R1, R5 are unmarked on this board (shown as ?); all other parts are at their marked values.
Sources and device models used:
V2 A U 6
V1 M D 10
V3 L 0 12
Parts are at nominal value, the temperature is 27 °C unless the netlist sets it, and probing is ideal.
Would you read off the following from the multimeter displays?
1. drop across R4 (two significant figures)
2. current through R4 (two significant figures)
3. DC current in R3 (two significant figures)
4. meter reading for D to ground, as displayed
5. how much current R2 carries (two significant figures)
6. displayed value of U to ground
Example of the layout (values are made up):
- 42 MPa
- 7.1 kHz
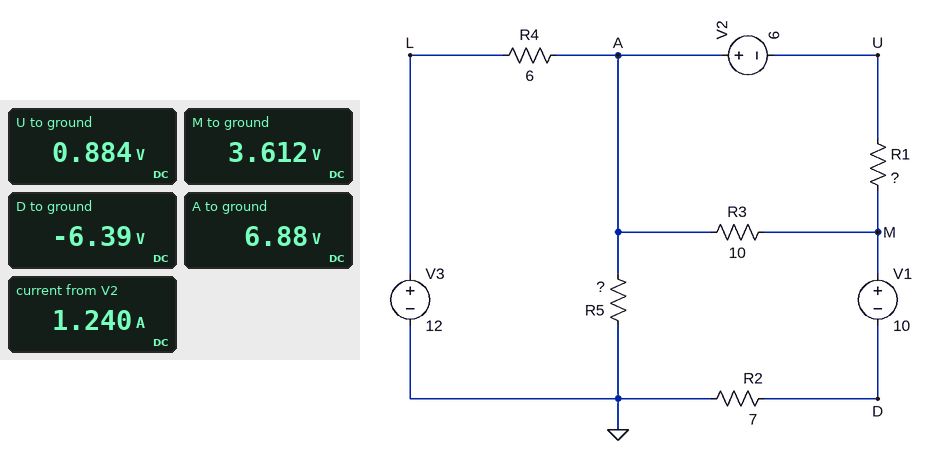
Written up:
- 5.1 V
- 850 mA
- 330 mA
- -6.39 V
- 910 mA
- 0.884 V
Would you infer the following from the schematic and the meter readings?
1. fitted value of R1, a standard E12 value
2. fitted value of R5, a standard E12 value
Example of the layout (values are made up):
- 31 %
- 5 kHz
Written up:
- 2.2 Ω
- 3.9 Ω
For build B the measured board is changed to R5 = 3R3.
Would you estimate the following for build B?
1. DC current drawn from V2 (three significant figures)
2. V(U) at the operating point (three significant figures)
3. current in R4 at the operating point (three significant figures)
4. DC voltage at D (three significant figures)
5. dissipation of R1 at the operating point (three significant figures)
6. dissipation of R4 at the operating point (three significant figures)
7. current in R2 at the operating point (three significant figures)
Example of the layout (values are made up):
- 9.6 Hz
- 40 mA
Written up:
- 1.29 A
- 334 mV
- 944 mA
- -6.83 V
- 3.67 W
- 5.35 W
- 975 mA
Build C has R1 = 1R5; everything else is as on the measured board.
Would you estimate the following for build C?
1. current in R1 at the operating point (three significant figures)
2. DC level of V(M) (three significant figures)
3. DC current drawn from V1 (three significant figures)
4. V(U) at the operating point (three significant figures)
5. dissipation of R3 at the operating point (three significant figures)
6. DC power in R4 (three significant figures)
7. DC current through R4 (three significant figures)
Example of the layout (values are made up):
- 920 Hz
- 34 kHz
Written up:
- 1.38 A
- 3.12 V
- 983 mA
- 1.05 V
- 1.55 W
- 4.08 W
- 825 mA
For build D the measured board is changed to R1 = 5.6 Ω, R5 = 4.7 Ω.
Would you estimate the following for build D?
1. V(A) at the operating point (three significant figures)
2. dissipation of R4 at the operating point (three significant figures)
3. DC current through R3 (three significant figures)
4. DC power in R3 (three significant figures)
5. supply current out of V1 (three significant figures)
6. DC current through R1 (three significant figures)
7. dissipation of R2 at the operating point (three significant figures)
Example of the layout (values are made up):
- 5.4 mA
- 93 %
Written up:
- 6.98 V
- 4.20 W
- 152 mA
- 231 mW
- 648 mA
- 800 mA
- 2.94 W
